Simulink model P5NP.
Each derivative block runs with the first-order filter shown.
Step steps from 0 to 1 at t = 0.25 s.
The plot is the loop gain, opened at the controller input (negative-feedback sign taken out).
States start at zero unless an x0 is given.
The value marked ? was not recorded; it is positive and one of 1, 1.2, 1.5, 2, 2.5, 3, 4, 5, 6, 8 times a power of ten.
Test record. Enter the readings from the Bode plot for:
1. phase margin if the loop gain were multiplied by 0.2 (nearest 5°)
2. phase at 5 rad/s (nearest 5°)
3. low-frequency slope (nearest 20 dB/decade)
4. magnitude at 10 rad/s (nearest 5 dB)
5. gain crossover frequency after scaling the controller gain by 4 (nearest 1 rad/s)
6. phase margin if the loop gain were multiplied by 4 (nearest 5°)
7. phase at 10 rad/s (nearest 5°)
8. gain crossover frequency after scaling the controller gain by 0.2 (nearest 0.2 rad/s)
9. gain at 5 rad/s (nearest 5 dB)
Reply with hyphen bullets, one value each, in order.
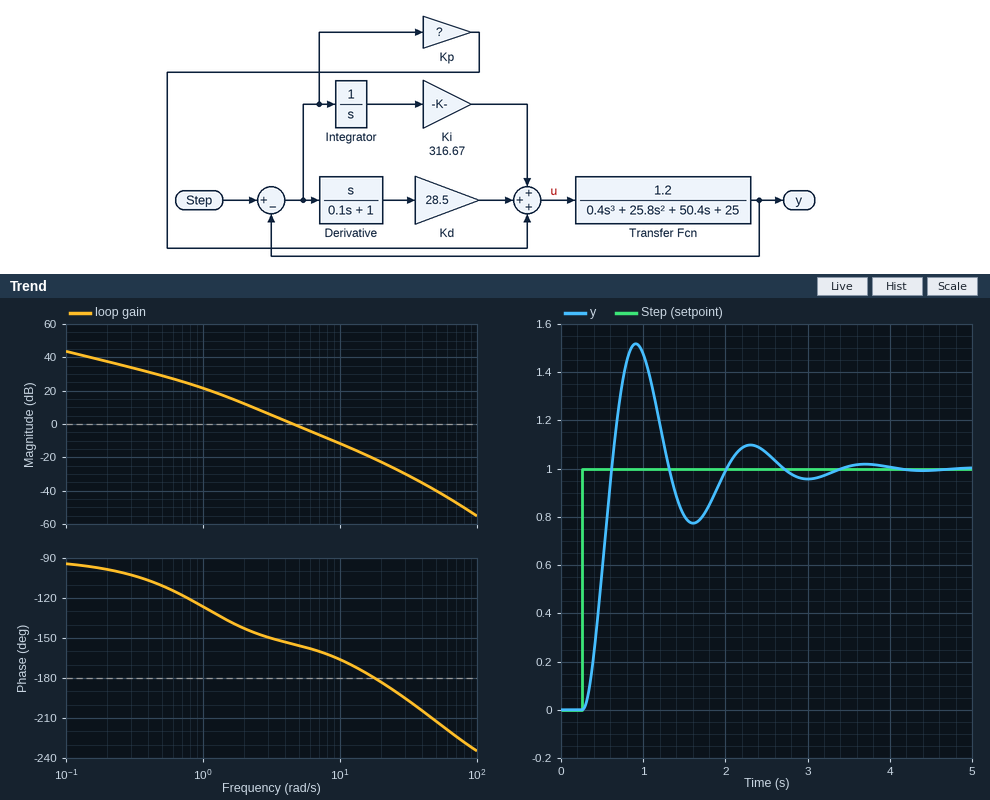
- 40°
- -155°
- -20 dB/decade
- -10 dB
- 10 rad/s
- 15°
- -165°
- 1.8 rad/s
- 0 dB
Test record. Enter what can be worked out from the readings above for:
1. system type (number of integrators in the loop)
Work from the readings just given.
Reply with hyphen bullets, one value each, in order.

- 1
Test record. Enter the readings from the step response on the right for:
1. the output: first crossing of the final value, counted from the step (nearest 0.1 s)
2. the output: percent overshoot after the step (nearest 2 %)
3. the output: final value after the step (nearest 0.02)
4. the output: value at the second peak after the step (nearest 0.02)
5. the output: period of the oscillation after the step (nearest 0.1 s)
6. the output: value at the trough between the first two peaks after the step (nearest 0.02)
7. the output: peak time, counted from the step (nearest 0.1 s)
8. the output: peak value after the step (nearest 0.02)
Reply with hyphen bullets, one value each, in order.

- 0.4 s
- 52 %
- 1.00
- 1.10
- 1.4 s
- 0.78
- 0.7 s
- 1.52
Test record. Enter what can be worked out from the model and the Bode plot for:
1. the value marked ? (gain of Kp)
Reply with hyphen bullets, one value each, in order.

- 400
